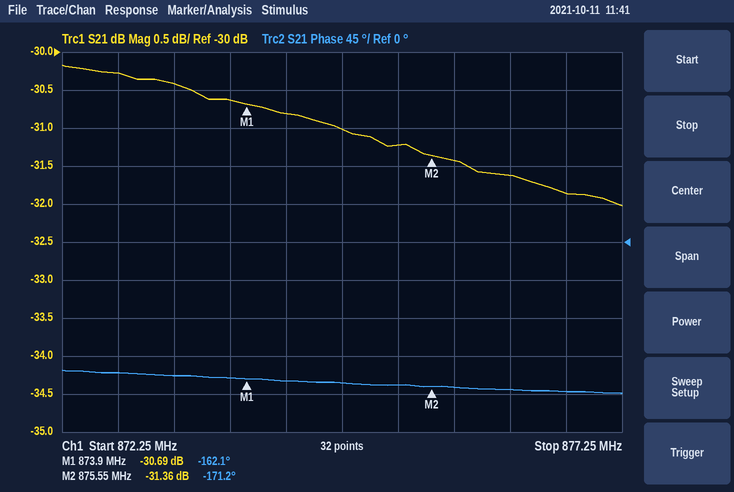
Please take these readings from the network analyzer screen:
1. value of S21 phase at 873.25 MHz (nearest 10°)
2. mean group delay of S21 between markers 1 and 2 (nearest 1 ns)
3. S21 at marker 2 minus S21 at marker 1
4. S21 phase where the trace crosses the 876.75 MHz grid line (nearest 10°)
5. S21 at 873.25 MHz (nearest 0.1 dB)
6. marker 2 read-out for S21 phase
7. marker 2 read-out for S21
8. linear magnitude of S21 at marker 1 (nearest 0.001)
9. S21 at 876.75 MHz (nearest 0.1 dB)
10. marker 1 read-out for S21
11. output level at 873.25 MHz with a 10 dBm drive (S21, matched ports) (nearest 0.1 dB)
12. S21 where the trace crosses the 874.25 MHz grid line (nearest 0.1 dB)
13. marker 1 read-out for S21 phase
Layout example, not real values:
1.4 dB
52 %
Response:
-160°
15 ns
-0.67 dB
-180°
-30.4 dB
-171.2°
-31.36 dB
0.029
-31.9 dB
-30.69 dB
-20.4 dBm
-30.8 dB
-162.1°
